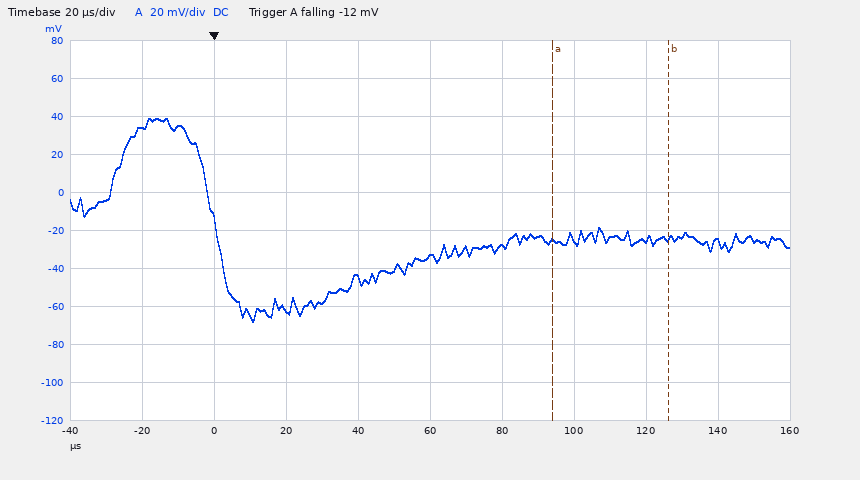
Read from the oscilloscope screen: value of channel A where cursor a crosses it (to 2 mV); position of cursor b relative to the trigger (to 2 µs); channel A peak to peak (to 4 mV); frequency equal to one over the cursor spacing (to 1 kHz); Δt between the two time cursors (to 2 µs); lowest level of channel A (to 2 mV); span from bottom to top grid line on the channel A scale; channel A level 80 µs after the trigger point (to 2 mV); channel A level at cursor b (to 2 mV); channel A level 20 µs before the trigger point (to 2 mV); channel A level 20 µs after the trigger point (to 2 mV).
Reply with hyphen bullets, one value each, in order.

- -26 mV
- +126 µs
- 108 mV
- 31 kHz
- 32 µs
- -68 mV
- 200 mV
- -28 mV
- -24 mV
- 34 mV
- -62 mV
